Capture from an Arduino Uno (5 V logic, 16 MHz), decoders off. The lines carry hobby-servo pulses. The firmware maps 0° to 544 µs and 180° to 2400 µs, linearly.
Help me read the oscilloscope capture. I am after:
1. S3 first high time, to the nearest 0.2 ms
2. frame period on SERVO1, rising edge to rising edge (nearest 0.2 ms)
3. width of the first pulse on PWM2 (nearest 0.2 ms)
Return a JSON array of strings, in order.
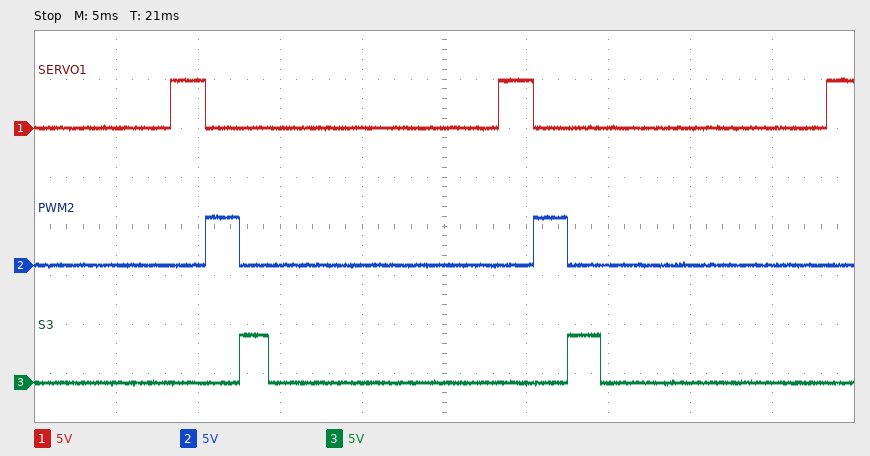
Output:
["1.8 ms", "20.0 ms", "2.0 ms"]
